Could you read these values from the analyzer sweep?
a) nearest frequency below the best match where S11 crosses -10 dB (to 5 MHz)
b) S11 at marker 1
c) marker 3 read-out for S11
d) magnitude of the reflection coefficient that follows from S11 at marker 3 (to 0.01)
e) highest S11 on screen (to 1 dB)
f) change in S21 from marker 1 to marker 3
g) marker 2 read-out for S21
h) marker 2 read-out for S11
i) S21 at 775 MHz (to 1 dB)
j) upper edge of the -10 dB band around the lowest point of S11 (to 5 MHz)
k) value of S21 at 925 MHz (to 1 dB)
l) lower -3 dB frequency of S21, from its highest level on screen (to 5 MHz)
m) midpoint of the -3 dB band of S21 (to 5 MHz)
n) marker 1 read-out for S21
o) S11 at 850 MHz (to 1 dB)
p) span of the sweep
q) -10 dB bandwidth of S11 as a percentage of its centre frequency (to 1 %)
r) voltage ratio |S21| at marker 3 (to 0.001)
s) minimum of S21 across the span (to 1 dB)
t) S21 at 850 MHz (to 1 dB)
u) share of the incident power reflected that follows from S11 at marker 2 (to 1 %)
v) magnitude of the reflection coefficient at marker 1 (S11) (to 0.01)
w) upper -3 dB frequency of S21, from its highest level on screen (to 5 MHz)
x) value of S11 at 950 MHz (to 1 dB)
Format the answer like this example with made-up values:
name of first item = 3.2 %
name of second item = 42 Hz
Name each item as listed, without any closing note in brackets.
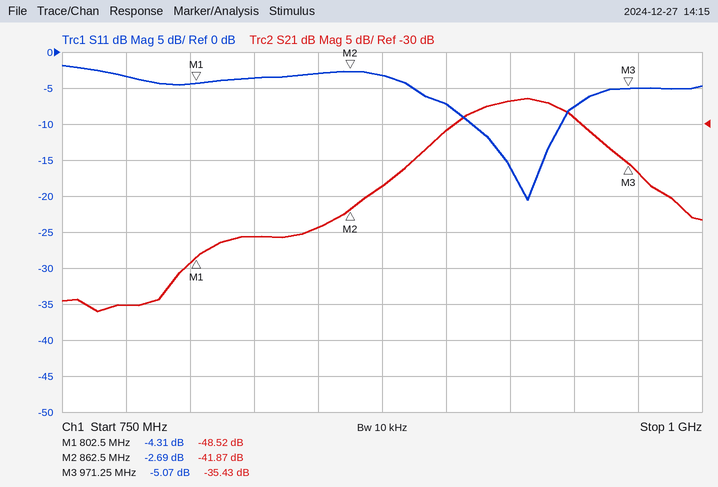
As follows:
nearest frequency below the best match where S11 crosses -10 dB = 910 MHz
S11 at marker 1 = -4.31 dB
marker 3 read-out for S11 = -5.07 dB
magnitude of the reflection coefficient that follows from S11 at marker 3 = 0.56
highest S11 on screen = -2 dB
change in S21 from marker 1 to marker 3 = 13.09 dB
marker 2 read-out for S21 = -41.87 dB
marker 2 read-out for S11 = -2.69 dB
S21 at 775 MHz = -55 dB
upper edge of the -10 dB band around the lowest point of S11 = 945 MHz
value of S21 at 925 MHz = -27 dB
lower -3 dB frequency of S21, from its highest level on screen = 905 MHz
midpoint of the -3 dB band of S21 = 930 MHz
marker 1 read-out for S21 = -48.52 dB
S11 at 850 MHz = -3 dB
span of the sweep = 250 MHz
-10 dB bandwidth of S11 as a percentage of its centre frequency = 4 %
voltage ratio |S21| at marker 3 = 0.017
minimum of S21 across the span = -56 dB
S21 at 850 MHz = -44 dB
share of the incident power reflected that follows from S11 at marker 2 = 54 %
magnitude of the reflection coefficient at marker 1 (S11) = 0.61
upper -3 dB frequency of S21, from its highest level on screen = 950 MHz
value of S11 at 950 MHz = -8 dB
